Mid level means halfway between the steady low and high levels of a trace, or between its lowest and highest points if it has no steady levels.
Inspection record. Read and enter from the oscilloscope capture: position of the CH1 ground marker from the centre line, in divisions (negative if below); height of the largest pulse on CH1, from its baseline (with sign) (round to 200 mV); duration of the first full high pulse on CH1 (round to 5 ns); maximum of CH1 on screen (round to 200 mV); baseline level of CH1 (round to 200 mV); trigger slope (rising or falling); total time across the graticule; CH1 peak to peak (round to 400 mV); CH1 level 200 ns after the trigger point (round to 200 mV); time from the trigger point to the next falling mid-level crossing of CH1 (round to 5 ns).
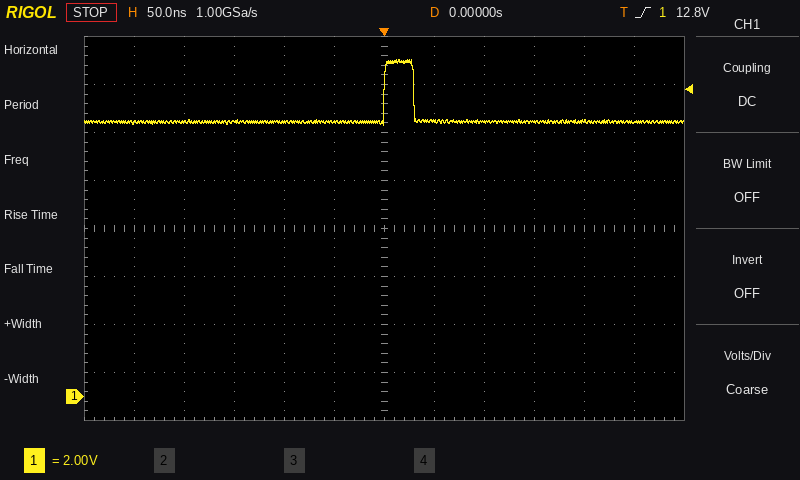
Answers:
-3.5 div
+2.6 V
30 ns
14.0 V
11.4 V
rising
600 ns
2.8 V
11.4 V
30 ns
